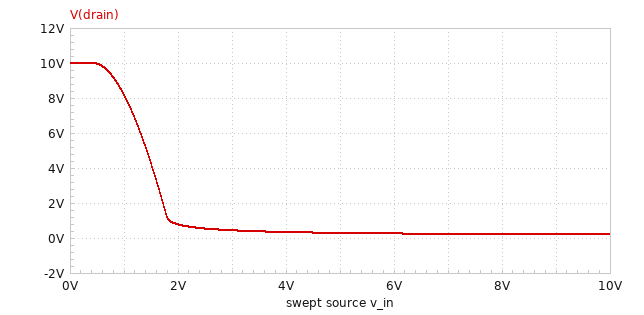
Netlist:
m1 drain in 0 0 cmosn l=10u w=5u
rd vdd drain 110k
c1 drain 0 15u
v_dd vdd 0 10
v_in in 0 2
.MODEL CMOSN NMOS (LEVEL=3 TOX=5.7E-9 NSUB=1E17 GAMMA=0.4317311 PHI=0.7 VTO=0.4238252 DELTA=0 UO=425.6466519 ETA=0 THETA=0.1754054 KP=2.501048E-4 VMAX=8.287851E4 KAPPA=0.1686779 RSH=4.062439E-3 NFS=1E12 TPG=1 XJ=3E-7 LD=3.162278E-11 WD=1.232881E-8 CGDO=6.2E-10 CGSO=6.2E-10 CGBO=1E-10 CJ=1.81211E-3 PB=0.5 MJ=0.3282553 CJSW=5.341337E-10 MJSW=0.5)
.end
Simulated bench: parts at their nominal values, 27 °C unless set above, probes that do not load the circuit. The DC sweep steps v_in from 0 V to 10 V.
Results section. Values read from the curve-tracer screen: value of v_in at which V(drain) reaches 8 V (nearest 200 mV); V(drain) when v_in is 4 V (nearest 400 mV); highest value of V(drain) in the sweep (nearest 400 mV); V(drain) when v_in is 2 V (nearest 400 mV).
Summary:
1.0 V
400 mV
10.0 V
800 mV
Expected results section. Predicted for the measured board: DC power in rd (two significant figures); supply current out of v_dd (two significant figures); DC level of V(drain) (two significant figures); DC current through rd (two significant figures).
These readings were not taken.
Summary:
770 µW
84 µA
780 mV
84 µA
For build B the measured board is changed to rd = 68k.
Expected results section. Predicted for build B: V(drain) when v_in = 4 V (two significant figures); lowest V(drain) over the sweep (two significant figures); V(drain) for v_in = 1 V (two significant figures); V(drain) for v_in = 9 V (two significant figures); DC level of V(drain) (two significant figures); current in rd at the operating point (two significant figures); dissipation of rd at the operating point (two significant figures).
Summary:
570 mV
330 mV
8.9 V
340 mV
3.0 V
100 µA
710 µW
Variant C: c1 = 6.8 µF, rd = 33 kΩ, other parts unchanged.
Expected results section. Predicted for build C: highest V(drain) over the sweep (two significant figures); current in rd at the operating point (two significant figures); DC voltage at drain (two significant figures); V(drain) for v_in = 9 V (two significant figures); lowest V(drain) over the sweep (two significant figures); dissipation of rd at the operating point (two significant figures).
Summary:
10 V
100 µA
6.6 V
700 mV
670 mV
350 µW
